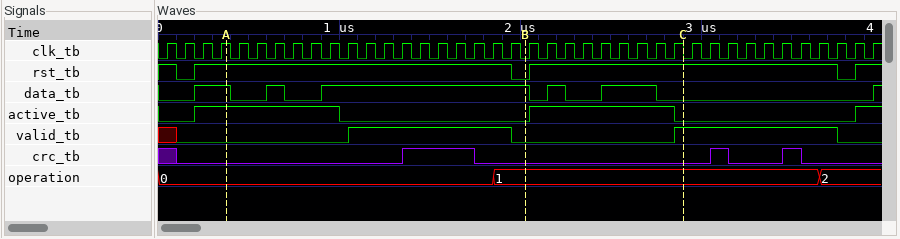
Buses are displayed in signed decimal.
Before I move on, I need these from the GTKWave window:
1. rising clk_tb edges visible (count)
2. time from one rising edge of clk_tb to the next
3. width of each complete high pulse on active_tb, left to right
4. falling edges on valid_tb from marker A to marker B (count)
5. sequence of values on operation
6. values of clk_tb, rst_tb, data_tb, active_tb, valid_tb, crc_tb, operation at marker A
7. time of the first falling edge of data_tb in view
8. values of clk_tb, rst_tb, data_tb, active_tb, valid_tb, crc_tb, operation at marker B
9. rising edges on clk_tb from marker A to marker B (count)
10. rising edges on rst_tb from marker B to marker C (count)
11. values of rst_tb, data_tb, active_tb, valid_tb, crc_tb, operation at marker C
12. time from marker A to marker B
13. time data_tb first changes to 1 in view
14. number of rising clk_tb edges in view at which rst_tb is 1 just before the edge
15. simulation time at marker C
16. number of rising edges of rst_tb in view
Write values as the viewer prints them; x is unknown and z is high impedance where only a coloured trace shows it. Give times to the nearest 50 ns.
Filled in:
40
100 ns
800 ns, 800 ns
1
0, 1, 2
clk_tb=1, rst_tb=1, data_tb=1, active_tb=1, valid_tb=0, crc_tb=0, operation=0
400 ns
clk_tb=0, rst_tb=0, data_tb=1, active_tb=0, valid_tb=0, crc_tb=0, operation=1
16
1
rst_tb=1, data_tb=0, active_tb=0, valid_tb=1, crc_tb=0, operation=1
1650 ns
200 ns
37
2900 ns
3
